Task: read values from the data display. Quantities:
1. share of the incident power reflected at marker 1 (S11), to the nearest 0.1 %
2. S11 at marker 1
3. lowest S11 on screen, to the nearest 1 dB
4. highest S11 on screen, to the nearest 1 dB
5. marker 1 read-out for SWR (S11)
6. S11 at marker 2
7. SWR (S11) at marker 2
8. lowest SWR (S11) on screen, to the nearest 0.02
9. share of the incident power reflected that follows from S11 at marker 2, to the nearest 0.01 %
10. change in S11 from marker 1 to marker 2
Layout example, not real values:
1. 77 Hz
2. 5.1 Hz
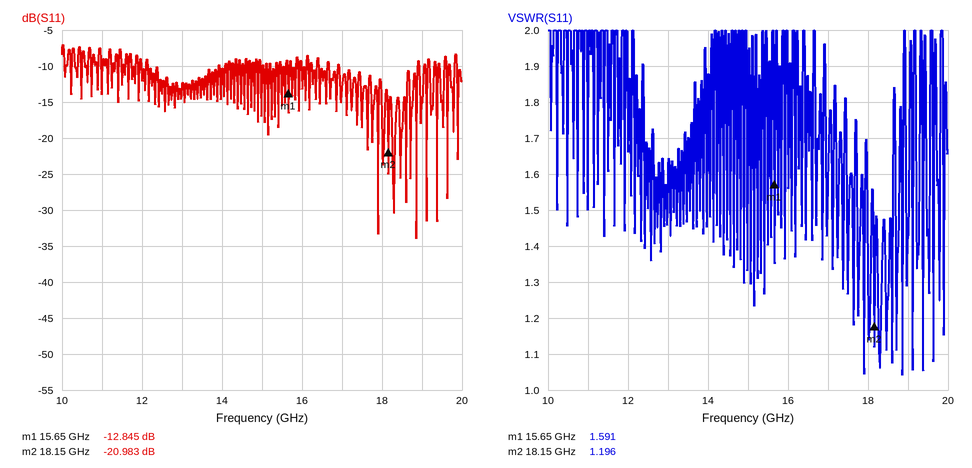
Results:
1. 5.2 %
2. -12.845 dB
3. -34 dB
4. -7 dB
5. 1.591
6. -20.983 dB
7. 1.196
8. 1.04
9. 0.80 %
10. -8.138 dB
